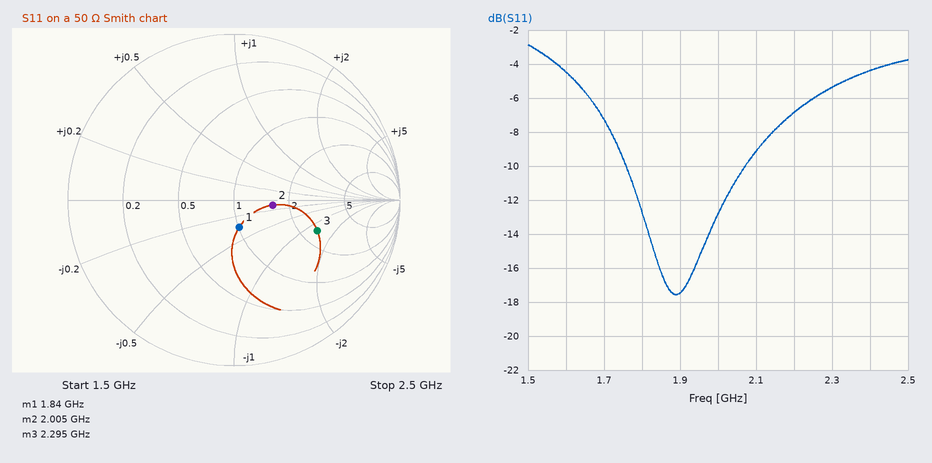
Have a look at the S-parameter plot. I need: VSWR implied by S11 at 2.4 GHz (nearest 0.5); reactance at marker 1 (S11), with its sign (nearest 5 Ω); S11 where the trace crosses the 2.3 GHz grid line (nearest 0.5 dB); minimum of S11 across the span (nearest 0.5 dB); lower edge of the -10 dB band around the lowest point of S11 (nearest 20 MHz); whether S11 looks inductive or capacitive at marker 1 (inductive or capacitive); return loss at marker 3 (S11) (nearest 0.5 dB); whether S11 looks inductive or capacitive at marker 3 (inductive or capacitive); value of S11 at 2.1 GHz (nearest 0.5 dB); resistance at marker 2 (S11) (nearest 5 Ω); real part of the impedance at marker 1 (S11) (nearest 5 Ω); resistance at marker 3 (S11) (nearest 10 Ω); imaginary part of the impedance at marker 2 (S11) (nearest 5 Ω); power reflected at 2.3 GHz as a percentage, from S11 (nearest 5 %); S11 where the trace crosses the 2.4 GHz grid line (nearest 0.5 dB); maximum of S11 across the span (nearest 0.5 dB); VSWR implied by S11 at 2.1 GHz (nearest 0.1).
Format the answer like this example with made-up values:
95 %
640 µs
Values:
4.0
-15 Ω
-5.5 dB
-17.5 dB
1.76 GHz
capacitive
5.5 dB
capacitive
-9.0 dB
80 Ω
50 Ω
130 Ω
-5 Ω
30 %
-4.5 dB
-3.0 dB
2.1
